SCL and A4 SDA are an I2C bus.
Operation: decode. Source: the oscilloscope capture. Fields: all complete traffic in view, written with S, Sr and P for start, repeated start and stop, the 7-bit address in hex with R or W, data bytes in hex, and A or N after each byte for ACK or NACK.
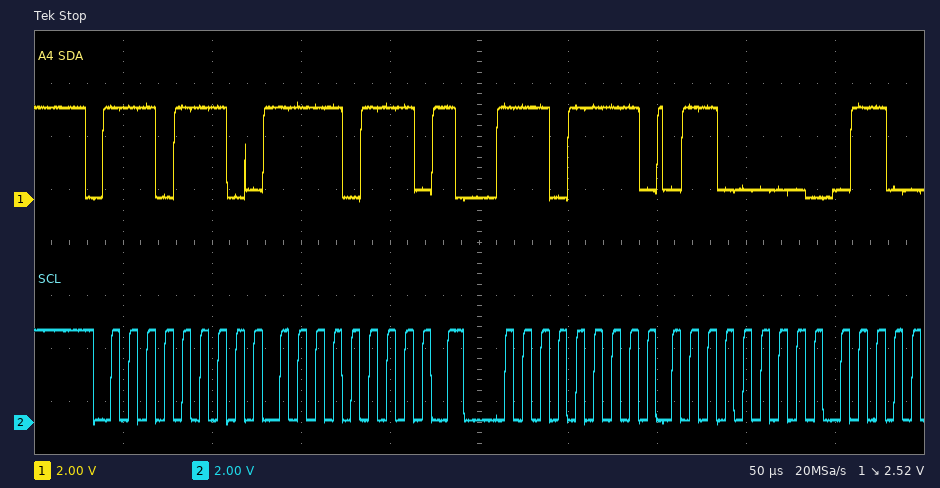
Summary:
S 77W A F7 A Sr 77R A 60 A
